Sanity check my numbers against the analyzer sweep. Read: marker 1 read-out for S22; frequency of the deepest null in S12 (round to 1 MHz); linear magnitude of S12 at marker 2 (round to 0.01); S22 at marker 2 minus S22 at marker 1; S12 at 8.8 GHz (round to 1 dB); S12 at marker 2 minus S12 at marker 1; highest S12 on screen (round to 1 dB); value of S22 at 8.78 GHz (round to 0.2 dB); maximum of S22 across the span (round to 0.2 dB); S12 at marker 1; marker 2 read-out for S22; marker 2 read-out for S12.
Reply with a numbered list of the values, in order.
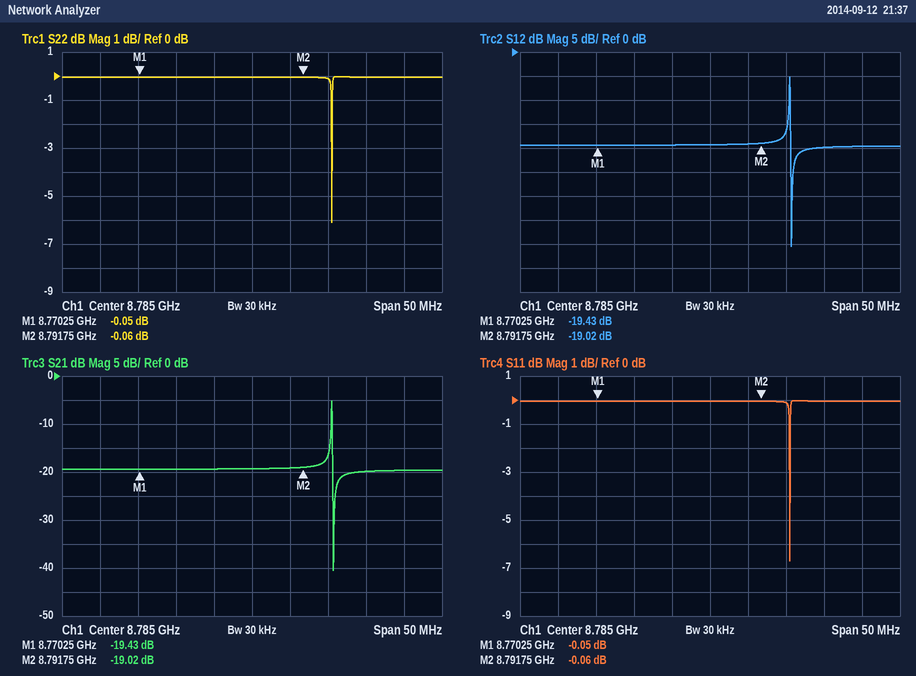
1. -0.05 dB
2. 8.796 GHz
3. 0.11
4. -0.01 dB
5. -20 dB
6. 0.41 dB
7. -5 dB
8. 0.0 dB
9. 0.0 dB
10. -19.43 dB
11. -0.06 dB
12. -19.02 dB
